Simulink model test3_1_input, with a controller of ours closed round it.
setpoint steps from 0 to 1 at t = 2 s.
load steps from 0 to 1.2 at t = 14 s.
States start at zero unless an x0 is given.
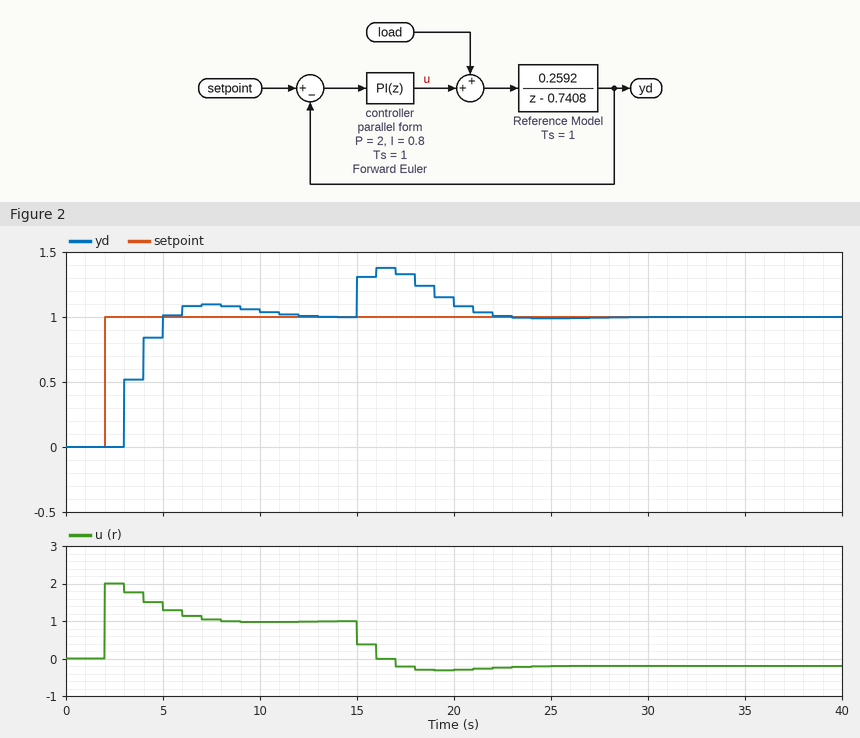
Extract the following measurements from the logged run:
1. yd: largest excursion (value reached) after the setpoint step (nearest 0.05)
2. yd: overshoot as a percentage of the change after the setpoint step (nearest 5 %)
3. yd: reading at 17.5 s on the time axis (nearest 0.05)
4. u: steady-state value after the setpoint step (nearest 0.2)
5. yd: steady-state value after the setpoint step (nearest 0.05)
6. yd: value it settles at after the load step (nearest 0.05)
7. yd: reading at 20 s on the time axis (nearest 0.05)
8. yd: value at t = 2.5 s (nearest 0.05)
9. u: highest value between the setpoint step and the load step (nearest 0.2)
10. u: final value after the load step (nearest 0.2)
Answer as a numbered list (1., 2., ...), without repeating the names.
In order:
1. 1.10
2. 10 %
3. 1.35
4. 1.0
5. 1.00
6. 1.00
7. 1.10
8. 0.00
9. 2.0
10. -0.2
